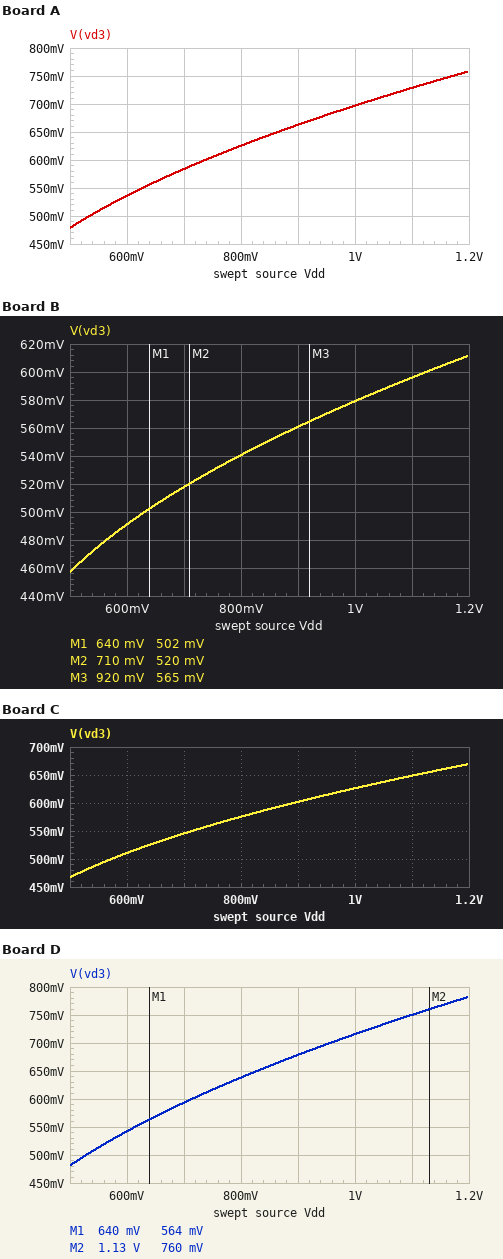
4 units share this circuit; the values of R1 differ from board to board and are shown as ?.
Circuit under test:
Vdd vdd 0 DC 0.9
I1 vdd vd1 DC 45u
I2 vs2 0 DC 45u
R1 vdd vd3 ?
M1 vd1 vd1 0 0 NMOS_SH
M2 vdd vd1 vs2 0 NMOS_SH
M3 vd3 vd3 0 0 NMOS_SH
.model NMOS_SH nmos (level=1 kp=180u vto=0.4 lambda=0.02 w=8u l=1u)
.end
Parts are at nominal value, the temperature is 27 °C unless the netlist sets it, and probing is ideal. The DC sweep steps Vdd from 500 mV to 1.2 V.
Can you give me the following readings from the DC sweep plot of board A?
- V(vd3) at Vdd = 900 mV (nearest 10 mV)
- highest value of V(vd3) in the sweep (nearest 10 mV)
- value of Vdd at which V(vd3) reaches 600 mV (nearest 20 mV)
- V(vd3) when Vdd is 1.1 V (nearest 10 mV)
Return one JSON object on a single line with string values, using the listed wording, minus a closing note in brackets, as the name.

{"V(vd3) at Vdd = 900 mV": "660 mV", "highest value of V(vd3) in the sweep": "760 mV", "value of Vdd at which V(vd3) reaches 600 mV": "740 mV", "V(vd3) when Vdd is 1.1 V": "730 mV"}
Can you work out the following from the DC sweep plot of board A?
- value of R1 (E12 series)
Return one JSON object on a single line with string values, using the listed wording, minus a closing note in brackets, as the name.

{"value of R1": "4.7 kΩ"}
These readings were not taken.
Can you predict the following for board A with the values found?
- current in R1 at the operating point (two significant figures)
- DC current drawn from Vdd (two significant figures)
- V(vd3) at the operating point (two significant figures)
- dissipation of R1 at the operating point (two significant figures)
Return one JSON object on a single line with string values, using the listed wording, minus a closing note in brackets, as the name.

{"current in R1 at the operating point": "50 µA", "DC current drawn from Vdd": "140 µA", "V(vd3) at the operating point": "660 mV", "dissipation of R1 at the operating point": "12 µW"}
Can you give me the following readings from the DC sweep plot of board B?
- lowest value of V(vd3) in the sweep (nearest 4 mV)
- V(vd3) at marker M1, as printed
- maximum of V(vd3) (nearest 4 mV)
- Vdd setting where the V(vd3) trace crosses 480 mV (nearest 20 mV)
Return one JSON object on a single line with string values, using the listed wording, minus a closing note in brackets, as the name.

{"lowest value of V(vd3) in the sweep": "456 mV", "V(vd3) at marker M1, as printed": "502 mV", "maximum of V(vd3)": "612 mV", "Vdd setting where the V(vd3) trace crosses 480 mV": "560 mV"}
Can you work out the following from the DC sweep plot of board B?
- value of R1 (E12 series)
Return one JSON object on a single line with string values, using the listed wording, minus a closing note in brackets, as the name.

{"value of R1": "18 kΩ"}
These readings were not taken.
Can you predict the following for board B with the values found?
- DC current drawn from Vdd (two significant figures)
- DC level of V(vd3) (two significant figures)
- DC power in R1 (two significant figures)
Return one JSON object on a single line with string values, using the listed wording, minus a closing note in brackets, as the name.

{"DC current drawn from Vdd": "110 µA", "DC level of V(vd3)": "560 mV", "DC power in R1": "6.4 µW"}
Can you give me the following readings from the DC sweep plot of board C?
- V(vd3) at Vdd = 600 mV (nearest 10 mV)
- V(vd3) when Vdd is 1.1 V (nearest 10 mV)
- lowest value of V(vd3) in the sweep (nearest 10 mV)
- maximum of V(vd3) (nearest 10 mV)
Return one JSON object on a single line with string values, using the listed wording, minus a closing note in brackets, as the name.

{"V(vd3) at Vdd = 600 mV": "510 mV", "V(vd3) when Vdd is 1.1 V": "650 mV", "lowest value of V(vd3) in the sweep": "470 mV", "maximum of V(vd3)": "670 mV"}
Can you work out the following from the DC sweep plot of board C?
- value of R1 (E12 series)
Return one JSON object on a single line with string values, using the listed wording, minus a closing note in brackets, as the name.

{"value of R1": "10 kΩ"}
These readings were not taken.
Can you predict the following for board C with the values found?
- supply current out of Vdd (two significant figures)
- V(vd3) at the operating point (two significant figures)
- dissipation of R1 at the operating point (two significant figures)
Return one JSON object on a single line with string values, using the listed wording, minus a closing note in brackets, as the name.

{"supply current out of Vdd": "120 µA", "V(vd3) at the operating point": "600 mV", "dissipation of R1 at the operating point": "8.9 µW"}
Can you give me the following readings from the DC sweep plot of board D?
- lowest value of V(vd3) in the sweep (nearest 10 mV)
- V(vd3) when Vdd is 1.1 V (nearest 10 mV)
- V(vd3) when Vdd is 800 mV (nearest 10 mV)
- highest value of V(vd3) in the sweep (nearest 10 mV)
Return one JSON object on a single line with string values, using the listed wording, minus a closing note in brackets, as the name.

{"lowest value of V(vd3) in the sweep": "480 mV", "V(vd3) when Vdd is 1.1 V": "750 mV", "V(vd3) when Vdd is 800 mV": "640 mV", "highest value of V(vd3) in the sweep": "780 mV"}
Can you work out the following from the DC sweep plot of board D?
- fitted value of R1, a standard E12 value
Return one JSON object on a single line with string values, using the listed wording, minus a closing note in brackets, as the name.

{"fitted value of R1, a standard E12 value": "3.9 kΩ"}
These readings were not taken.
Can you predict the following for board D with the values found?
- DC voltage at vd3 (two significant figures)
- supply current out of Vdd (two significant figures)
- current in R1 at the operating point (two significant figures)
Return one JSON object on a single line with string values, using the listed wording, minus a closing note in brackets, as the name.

{"DC voltage at vd3": "680 mV", "supply current out of Vdd": "150 µA", "current in R1 at the operating point": "57 µA"}
